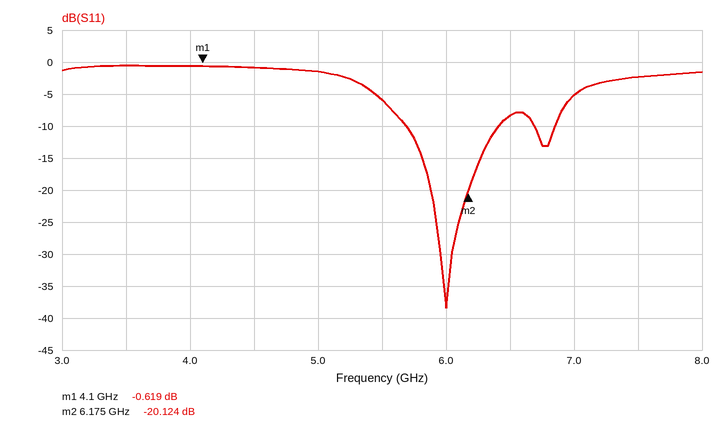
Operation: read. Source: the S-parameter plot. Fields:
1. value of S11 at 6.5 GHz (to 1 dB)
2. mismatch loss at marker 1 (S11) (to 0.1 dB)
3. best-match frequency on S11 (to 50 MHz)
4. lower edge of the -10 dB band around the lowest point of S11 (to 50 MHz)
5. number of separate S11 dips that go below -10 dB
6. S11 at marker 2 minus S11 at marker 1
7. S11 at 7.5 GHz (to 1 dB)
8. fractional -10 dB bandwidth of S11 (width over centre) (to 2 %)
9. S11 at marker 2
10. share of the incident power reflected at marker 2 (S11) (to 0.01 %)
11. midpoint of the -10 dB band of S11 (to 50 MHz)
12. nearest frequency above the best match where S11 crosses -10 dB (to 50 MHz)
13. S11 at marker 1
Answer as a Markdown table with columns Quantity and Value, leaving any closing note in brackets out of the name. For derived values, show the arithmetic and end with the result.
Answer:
| Quantity | Value |
|---|---|
| value of S11 at 6.5 GHz | -8 dB |
| mismatch loss at marker 1 (S11) | −10 log10(1 − 10^(-0.619/10)) ≈ 8.8 dB |
| best-match frequency on S11 | 6.00 GHz |
| lower edge of the -10 dB band around the lowest point of S11 | 5.70 GHz |
| number of separate S11 dips that go below -10 dB | 2 |
| S11 at marker 2 minus S11 at marker 1 | -20.124 − (-0.619) = -19.505 dB |
| S11 at 7.5 GHz | -2 dB |
| fractional -10 dB bandwidth of S11 (width over centre) | 700 MHz / 6.05 GHz ≈ 12 % |
| S11 at marker 2 | -20.124 dB |
| share of the incident power reflected at marker 2 (S11) | 10^(-20.124/10) ≈ 0.97 % |
| midpoint of the -10 dB band of S11 | 6.05 GHz |
| nearest frequency above the best match where S11 crosses -10 dB | 6.40 GHz |
| S11 at marker 1 | -0.619 dB |
